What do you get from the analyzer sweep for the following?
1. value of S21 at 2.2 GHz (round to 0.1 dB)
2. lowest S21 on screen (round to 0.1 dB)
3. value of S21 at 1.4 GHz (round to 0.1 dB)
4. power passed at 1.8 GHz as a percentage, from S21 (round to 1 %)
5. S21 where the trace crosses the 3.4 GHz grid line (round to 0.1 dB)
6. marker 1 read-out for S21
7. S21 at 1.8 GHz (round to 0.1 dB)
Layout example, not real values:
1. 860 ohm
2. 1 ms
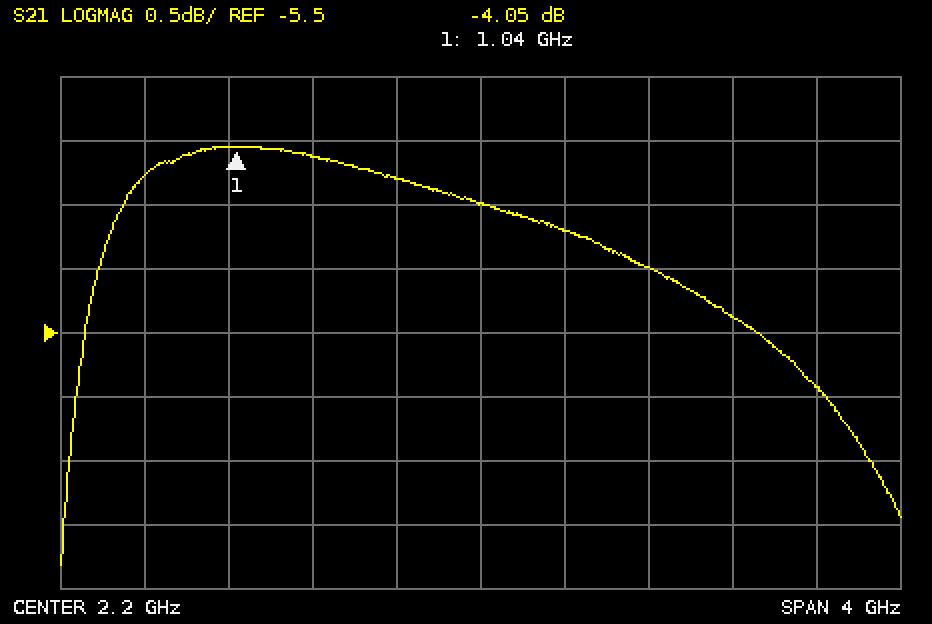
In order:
1. -4.5 dB
2. -7.3 dB
3. -4.1 dB
4. 37 %
5. -5.4 dB
6. -4.05 dB
7. -4.3 dB
